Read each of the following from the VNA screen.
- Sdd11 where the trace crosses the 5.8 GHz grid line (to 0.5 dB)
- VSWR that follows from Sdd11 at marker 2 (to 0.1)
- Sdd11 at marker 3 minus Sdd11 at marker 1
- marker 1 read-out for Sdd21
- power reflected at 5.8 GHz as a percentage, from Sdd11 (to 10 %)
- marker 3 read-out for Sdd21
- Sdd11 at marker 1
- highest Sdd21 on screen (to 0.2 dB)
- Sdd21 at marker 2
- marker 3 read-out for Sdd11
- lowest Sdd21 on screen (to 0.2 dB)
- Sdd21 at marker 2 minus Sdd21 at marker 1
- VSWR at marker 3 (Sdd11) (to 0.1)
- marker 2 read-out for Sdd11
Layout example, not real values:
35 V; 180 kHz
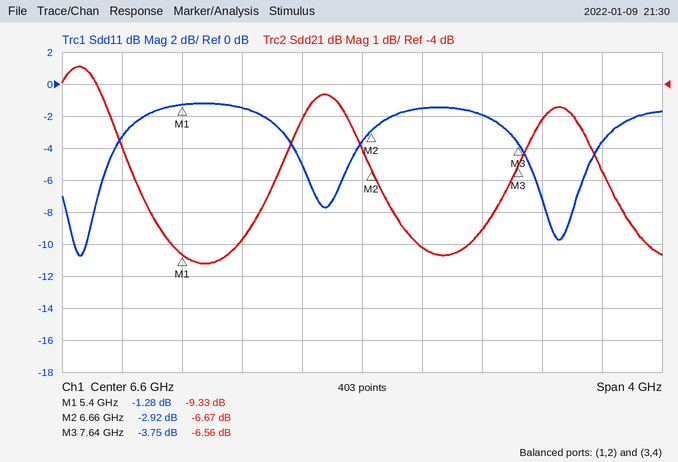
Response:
-1.5 dB; 6.0; -2.47 dB; -9.33 dB; 70 %; -6.56 dB; -1.28 dB; -3.4 dB; -6.67 dB; -3.75 dB; -9.6 dB; 2.66 dB; 4.7; -2.92 dB
